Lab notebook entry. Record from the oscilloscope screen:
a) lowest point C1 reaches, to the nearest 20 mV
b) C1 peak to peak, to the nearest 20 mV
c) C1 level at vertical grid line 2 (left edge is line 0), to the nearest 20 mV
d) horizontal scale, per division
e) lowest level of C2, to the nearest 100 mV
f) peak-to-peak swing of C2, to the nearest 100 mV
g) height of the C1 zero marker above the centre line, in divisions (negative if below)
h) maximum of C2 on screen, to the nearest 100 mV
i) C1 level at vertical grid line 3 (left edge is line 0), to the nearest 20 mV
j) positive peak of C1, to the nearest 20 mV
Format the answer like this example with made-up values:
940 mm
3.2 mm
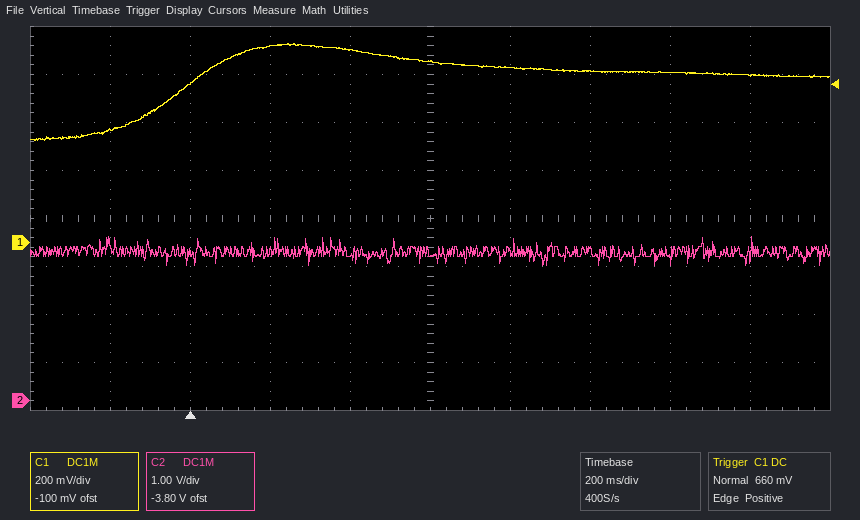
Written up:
420 mV
400 mV
660 mV
200 ms
2.8 V
600 mV
-0.5 div
3.4 V
820 mV
820 mV
